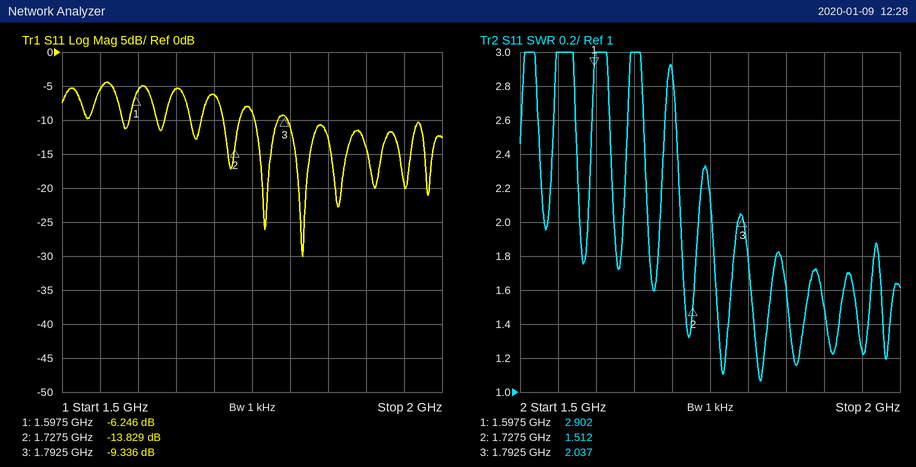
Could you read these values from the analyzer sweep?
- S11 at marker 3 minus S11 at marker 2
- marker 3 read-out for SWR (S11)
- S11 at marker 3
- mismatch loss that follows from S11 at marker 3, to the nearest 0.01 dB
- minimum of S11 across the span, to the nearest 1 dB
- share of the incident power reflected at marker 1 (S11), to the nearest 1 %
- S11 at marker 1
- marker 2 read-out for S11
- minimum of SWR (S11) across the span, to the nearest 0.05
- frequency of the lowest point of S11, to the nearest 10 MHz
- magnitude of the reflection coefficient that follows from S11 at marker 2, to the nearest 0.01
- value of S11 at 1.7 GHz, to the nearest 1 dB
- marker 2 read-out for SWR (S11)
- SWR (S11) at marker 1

4.493 dB
2.037
-9.336 dB
0.54 dB
-30 dB
24 %
-6.246 dB
-13.829 dB
1.05
1.82 GHz
0.20
-6 dB
1.512
2.902
